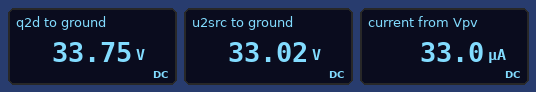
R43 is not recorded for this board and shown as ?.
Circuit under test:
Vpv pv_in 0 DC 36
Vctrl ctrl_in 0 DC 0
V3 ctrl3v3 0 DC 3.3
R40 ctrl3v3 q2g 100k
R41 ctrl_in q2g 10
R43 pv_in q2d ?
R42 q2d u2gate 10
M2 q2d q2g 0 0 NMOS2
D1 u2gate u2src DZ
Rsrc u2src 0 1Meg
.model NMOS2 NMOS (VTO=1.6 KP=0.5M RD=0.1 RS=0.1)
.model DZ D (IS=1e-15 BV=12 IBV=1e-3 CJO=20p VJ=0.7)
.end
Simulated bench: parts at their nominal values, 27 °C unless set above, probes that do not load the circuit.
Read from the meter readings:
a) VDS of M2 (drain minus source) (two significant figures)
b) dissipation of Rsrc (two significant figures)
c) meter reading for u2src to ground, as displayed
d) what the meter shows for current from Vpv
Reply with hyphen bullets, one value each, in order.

- 34 V
- 1.1 mW
- 33.02 V
- 33.0 µA
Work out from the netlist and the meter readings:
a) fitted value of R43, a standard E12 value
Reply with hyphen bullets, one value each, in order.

- 68 kΩ
